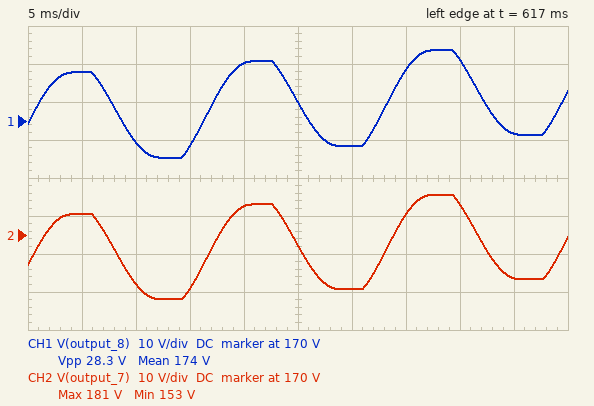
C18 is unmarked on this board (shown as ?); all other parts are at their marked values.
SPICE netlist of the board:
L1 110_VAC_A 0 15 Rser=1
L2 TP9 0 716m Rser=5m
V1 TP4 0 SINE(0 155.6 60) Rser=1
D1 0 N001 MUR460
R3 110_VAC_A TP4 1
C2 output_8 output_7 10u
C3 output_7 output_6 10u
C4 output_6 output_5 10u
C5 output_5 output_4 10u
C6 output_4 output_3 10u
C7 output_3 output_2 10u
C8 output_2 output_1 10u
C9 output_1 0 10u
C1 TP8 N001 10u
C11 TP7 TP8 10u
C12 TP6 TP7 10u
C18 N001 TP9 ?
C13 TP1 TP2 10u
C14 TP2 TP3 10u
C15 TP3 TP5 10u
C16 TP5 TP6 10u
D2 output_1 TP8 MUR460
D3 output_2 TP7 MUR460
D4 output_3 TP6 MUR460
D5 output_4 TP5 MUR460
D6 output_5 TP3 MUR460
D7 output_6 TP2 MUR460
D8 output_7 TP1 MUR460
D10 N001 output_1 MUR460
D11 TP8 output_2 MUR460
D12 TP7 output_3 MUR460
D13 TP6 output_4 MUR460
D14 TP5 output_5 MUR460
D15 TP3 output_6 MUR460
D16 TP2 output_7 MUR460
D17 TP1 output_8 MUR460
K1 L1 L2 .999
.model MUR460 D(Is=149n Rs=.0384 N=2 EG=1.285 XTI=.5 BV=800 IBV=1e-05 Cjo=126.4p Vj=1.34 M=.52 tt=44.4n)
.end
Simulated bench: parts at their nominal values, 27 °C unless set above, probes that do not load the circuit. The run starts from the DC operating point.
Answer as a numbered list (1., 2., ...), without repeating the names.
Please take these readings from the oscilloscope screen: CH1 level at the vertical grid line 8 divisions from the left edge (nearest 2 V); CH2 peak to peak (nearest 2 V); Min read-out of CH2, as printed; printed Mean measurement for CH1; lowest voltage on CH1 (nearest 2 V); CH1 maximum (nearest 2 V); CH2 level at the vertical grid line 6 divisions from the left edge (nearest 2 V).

1. 186 V
2. 28 V
3. 153 V
4. 174 V
5. 160 V
6. 188 V
7. 156 V
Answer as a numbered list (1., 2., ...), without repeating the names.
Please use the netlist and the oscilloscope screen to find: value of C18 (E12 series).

1. 3.3 µF
